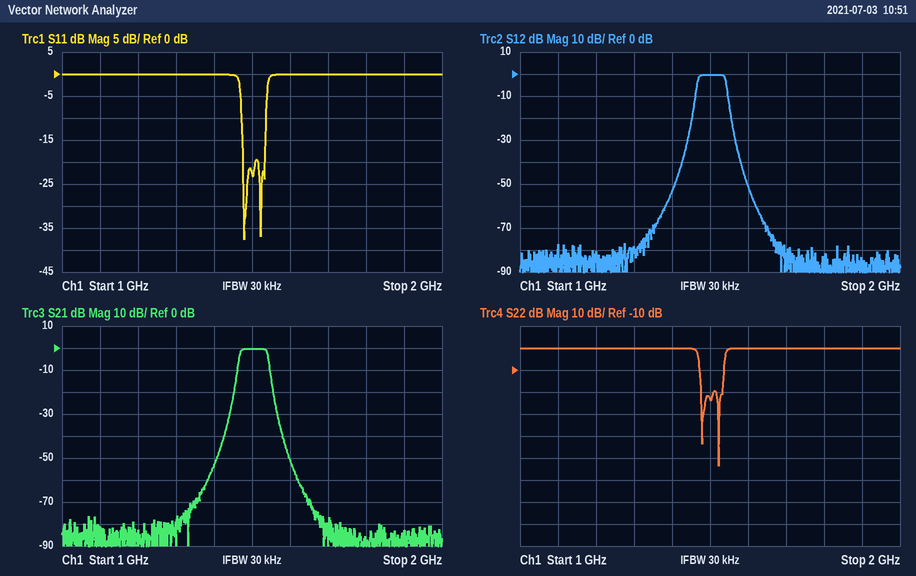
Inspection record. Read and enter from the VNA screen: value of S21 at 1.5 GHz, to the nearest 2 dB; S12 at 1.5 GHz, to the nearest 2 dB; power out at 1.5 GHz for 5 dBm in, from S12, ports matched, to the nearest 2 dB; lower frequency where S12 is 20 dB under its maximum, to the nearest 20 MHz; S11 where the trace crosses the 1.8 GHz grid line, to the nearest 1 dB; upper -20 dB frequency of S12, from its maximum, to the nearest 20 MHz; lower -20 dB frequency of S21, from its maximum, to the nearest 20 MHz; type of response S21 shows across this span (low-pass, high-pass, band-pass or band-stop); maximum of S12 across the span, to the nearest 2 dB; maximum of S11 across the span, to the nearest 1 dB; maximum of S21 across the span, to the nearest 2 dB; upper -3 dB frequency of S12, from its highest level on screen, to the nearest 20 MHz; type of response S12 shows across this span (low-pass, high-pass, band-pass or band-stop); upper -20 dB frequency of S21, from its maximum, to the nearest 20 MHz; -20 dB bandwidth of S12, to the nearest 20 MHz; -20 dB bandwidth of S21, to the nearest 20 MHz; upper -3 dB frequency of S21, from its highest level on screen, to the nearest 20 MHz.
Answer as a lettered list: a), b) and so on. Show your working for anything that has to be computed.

a) 0 dB
b) 0 dB
c) 5 dBm + (0 dB) = 4 dBm
d) 1.46 GHz
e) 0 dB
f) 1.56 GHz
g) 1.46 GHz
h) band-pass
i) 0 dB
j) 0 dB
k) 0 dB
l) 1.54 GHz
m) band-pass
n) 1.56 GHz
o) 1.56 GHz − 1.46 GHz = 100 MHz
p) 1.56 GHz − 1.46 GHz = 100 MHz
q) 1.54 GHz
